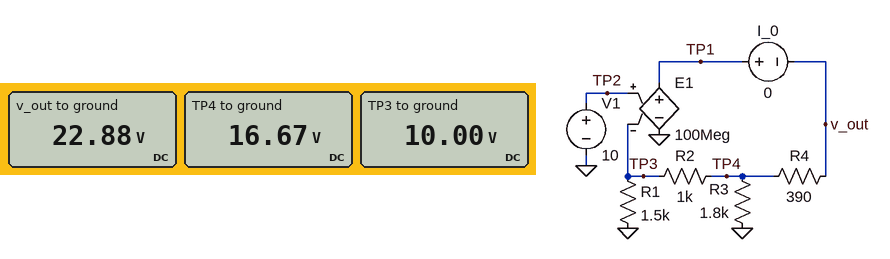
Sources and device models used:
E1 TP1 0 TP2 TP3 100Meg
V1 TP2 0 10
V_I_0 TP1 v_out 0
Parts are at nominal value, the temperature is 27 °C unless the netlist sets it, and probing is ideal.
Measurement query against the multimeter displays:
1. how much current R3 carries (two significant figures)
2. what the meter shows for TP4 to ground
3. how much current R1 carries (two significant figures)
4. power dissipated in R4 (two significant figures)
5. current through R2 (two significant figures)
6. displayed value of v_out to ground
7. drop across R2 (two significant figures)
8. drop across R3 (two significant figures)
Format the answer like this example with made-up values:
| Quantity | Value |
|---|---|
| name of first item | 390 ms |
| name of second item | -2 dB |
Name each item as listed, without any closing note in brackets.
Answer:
| Quantity | Value |
|---|---|
| how much current R3 carries | 9.3 mA |
| what the meter shows for TP4 to ground | 16.67 V |
| how much current R1 carries | 6.7 mA |
| power dissipated in R4 | 99 mW |
| current through R2 | 6.7 mA |
| displayed value of v_out to ground | 22.88 V |
| drop across R2 | 6.7 V |
| drop across R3 | 17 V |
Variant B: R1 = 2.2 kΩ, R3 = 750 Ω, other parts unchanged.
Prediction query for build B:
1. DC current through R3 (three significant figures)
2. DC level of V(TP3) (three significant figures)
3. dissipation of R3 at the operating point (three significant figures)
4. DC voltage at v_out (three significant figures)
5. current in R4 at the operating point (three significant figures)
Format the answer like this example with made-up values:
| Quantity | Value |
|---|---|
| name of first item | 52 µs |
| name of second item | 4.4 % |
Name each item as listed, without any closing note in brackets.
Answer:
| Quantity | Value |
|---|---|
| DC current through R3 | 19.4 mA |
| DC level of V(TP3) | 10.0 V |
| dissipation of R3 at the operating point | 282 mW |
| DC voltage at v_out | 23.9 V |
| current in R4 at the operating point | 23.9 mA |
